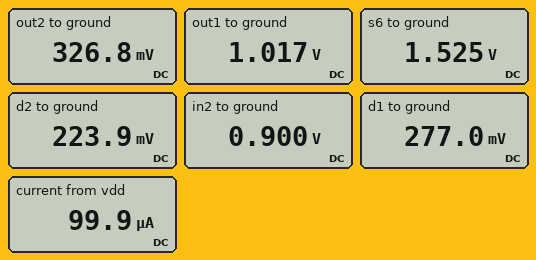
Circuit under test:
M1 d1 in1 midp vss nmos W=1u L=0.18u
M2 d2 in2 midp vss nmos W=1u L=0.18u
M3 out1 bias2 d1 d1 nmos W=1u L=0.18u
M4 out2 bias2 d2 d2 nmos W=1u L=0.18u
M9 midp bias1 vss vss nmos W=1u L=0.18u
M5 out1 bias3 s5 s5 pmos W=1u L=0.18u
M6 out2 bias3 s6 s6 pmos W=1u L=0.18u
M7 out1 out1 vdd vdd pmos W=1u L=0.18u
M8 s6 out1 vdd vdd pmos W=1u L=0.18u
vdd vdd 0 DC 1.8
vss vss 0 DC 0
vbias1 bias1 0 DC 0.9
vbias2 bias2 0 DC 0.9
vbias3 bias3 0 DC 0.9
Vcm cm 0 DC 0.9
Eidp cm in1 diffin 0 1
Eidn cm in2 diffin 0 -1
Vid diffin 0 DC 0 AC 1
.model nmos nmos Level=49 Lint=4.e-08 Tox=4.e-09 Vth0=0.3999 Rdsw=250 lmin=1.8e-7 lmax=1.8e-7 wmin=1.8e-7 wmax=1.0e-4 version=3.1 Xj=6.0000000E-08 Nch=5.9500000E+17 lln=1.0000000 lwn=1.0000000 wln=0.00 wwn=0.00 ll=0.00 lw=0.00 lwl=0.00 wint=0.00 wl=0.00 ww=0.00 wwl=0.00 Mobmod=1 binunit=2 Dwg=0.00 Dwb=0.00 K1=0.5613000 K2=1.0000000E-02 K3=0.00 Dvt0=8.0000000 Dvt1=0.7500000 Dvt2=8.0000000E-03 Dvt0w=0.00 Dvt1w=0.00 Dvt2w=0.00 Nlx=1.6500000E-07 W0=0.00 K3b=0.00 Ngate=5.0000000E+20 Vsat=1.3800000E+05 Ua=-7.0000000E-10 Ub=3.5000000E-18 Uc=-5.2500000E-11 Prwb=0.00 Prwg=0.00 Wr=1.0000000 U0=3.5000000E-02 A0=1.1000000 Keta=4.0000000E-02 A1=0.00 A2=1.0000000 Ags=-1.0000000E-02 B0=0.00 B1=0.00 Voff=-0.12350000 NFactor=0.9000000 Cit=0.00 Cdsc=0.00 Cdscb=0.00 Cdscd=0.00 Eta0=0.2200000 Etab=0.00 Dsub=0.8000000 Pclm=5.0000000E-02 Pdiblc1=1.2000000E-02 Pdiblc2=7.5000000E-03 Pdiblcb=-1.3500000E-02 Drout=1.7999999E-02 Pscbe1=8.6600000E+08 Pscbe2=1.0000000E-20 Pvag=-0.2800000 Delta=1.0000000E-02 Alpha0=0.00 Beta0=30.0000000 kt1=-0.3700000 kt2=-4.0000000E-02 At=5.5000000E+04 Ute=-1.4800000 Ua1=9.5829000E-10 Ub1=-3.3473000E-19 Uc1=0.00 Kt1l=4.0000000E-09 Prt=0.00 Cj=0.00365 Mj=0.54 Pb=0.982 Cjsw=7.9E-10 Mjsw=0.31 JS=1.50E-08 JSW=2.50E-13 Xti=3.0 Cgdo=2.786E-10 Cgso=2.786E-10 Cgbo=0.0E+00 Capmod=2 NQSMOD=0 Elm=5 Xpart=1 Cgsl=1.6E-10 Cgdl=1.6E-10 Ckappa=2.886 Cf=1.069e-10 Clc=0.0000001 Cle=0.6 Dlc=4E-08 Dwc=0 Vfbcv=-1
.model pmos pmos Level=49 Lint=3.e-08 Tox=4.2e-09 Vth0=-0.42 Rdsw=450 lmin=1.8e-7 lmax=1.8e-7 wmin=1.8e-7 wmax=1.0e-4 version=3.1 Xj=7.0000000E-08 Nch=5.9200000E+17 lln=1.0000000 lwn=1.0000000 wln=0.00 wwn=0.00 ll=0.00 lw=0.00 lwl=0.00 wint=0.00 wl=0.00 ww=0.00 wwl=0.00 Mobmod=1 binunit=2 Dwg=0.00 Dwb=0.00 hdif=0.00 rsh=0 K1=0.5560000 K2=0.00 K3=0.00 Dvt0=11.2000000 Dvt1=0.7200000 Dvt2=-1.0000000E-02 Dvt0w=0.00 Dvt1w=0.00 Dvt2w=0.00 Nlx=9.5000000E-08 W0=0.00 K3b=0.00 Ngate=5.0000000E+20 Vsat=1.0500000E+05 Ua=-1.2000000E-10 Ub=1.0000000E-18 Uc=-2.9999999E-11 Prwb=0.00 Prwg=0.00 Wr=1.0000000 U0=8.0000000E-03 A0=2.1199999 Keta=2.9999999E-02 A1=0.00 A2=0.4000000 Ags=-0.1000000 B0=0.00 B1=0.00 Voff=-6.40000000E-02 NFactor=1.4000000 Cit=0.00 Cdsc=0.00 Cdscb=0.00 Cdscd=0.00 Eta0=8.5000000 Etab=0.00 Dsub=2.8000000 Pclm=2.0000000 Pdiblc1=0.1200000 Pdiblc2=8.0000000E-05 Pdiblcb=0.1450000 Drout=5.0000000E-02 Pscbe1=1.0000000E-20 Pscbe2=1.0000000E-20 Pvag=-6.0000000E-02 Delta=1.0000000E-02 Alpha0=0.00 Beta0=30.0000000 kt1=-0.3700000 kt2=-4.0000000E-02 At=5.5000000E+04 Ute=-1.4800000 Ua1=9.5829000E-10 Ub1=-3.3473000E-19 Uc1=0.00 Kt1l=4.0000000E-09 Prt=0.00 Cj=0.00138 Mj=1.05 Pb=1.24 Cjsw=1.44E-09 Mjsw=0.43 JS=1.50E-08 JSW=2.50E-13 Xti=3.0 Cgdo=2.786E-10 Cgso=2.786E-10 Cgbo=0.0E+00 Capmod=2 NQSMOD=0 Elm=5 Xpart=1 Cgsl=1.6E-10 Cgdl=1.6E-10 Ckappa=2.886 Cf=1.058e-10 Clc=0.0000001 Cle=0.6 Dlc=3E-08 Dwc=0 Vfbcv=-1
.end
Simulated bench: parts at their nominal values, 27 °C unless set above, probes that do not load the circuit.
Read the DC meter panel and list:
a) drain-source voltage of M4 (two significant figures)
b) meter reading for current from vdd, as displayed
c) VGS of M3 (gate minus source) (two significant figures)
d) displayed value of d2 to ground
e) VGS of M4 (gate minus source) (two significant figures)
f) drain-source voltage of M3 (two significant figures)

100 mV
99.9 µA
620 mV
223.9 mV
680 mV
740 mV
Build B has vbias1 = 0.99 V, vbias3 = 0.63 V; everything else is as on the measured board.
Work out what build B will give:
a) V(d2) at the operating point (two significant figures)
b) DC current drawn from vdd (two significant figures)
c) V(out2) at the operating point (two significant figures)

240 mV
110 µA
430 mV
